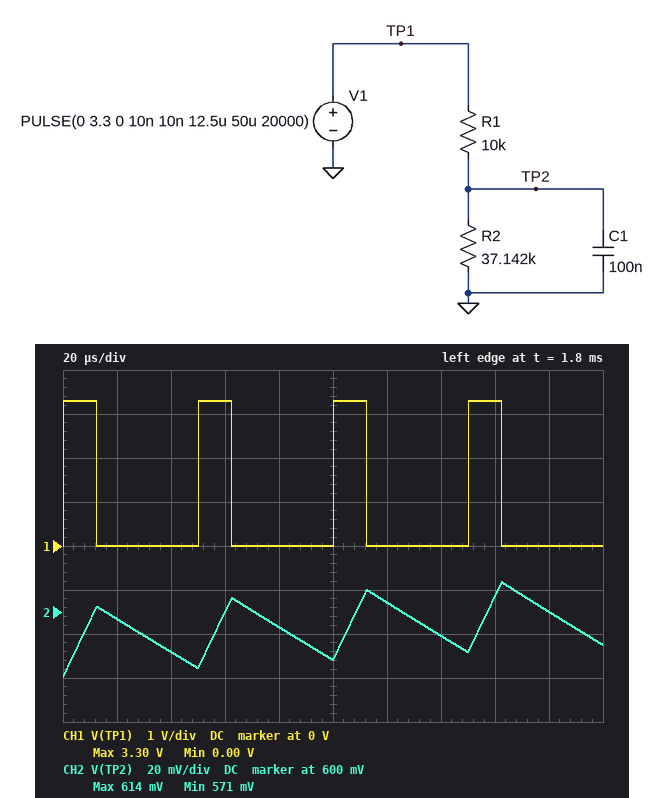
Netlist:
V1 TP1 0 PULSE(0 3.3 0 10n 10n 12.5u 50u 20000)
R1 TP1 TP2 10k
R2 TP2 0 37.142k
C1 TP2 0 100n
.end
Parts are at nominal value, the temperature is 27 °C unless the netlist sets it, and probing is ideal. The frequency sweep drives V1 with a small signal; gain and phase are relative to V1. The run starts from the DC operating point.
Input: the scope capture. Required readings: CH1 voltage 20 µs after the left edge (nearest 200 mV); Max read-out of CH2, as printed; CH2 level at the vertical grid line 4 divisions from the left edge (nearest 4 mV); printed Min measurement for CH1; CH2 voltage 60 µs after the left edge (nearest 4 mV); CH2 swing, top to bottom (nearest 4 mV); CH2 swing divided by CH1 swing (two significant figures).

0 V
614 mV
592 mV
0.00 V
600 mV
44 mV
0.013
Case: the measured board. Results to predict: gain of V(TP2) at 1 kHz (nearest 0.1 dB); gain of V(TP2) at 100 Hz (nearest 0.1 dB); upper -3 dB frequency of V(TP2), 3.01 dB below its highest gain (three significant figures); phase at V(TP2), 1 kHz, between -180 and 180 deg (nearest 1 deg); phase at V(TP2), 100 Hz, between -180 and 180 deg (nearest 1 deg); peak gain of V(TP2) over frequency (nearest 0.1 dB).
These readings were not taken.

-16.1 dB
-3.0 dB
202 Hz
-79 deg
-26 deg
-2.1 dB
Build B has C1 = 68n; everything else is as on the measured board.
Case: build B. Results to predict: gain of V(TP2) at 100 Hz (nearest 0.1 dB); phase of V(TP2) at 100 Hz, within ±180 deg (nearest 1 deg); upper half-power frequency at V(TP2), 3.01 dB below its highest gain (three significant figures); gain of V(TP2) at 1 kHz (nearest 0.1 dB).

-2.5 dB
-19 deg
297 Hz
-13.0 dB
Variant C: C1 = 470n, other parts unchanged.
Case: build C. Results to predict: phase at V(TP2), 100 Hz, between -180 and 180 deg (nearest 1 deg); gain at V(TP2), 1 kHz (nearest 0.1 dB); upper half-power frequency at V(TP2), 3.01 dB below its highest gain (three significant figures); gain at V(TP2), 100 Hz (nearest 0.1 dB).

-67 deg
-29.4 dB
43.0 Hz
-10.1 dB
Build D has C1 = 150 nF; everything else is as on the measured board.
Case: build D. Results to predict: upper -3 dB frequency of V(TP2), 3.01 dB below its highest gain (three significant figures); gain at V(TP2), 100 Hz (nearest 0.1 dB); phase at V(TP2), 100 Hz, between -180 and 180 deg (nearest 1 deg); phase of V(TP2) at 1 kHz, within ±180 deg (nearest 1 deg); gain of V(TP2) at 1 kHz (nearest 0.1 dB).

135 Hz
-4.0 dB
-37 deg
-82 deg
-19.6 dB
